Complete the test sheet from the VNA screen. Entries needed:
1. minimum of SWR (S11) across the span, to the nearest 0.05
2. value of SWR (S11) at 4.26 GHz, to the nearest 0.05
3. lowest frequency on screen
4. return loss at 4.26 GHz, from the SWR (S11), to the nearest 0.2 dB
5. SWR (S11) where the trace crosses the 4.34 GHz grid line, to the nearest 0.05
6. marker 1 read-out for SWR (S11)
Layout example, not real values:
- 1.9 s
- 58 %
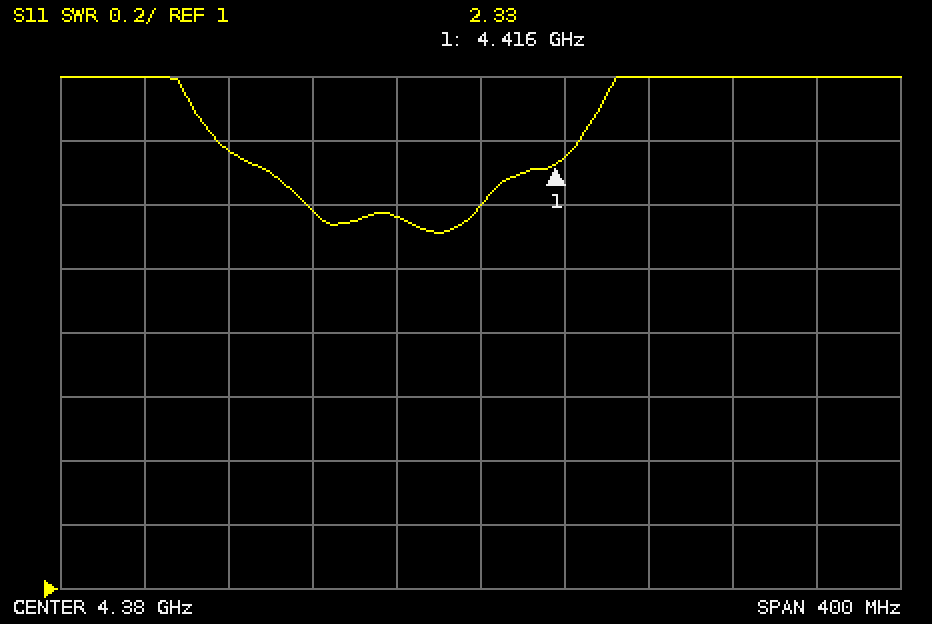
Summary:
- 2.10
- 2.35
- 4.18 GHz
- 7.8 dB
- 2.15
- 2.33
